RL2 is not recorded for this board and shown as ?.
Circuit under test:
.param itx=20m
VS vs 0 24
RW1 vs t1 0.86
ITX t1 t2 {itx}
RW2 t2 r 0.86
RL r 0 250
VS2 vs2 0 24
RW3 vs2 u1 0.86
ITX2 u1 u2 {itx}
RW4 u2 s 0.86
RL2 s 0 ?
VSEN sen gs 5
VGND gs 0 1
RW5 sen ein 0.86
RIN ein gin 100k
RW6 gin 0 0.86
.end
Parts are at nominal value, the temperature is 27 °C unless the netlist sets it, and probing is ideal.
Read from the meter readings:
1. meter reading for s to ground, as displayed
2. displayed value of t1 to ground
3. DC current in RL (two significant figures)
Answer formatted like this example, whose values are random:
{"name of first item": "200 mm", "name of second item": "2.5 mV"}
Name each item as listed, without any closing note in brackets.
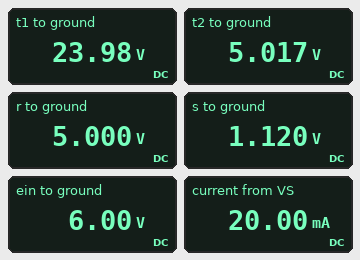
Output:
{"meter reading for s to ground, as displayed": "1.120 V", "displayed value of t1 to ground": "23.98 V", "DC current in RL": "20 mA"}
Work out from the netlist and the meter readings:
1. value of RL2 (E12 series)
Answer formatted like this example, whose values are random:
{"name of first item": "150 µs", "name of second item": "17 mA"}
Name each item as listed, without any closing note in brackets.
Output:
{"value of RL2": "56 Ω"}
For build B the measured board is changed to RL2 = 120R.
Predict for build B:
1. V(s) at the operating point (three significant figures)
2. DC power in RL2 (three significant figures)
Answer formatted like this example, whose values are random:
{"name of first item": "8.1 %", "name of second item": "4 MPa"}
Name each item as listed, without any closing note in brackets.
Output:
{"V(s) at the operating point": "2.40 V", "DC power in RL2": "48.0 mW"}
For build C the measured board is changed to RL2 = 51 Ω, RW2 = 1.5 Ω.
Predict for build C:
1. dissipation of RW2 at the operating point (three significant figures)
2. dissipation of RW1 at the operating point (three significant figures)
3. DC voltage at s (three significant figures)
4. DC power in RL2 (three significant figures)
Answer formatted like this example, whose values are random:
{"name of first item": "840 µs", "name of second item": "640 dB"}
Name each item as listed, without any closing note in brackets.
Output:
{"dissipation of RW2 at the operating point": "600 µW", "dissipation of RW1 at the operating point": "344 µW", "DC voltage at s": "1.02 V", "DC power in RL2": "20.4 mW"}
